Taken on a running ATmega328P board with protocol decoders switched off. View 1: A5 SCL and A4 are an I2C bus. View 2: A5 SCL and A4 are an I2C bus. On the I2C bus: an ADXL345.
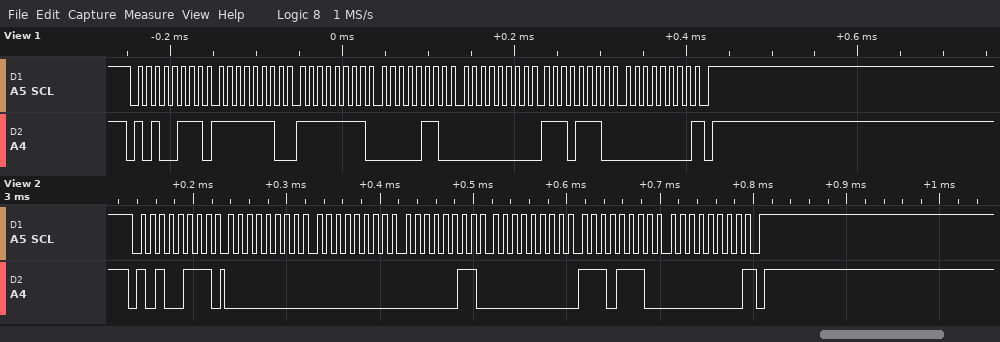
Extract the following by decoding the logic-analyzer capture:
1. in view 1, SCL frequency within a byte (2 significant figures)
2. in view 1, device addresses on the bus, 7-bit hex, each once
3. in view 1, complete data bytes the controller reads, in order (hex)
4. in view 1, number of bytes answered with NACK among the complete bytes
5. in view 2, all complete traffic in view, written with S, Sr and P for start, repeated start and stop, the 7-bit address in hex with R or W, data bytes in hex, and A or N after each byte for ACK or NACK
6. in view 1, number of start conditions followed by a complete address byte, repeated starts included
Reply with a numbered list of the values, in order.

1. 100 kHz
2. 0x53
3. FE FF 06 00 EE 00
4. 1
5. S 53R A 00 A 00 A 03 A 00 A EE A 00 N P
6. 1
